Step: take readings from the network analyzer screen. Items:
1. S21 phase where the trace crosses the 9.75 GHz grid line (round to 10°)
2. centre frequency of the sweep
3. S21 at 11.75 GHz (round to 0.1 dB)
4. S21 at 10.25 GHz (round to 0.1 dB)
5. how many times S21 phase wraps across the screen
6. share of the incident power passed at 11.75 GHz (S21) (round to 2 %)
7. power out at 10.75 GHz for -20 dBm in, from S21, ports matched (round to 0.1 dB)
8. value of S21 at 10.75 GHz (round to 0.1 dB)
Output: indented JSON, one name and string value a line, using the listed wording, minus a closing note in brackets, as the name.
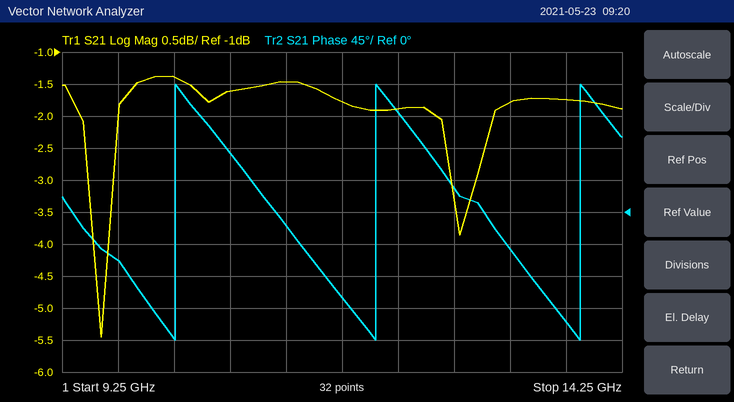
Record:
{
  "S21 phase where the trace crosses the 9.75 GHz grid line": "-70°",
  "centre frequency of the sweep": "11.75 GHz",
  "S21 at 11.75 GHz": "-1.8 dB",
  "S21 at 10.25 GHz": "-1.4 dB",
  "how many times S21 phase wraps across the screen": "3",
  "share of the incident power passed at 11.75 GHz (S21)": "66 %",
  "power out at 10.75 GHz for -20 dBm in, from S21, ports matched": "-21.6 dBm",
  "value of S21 at 10.75 GHz": "-1.6 dB"
}
